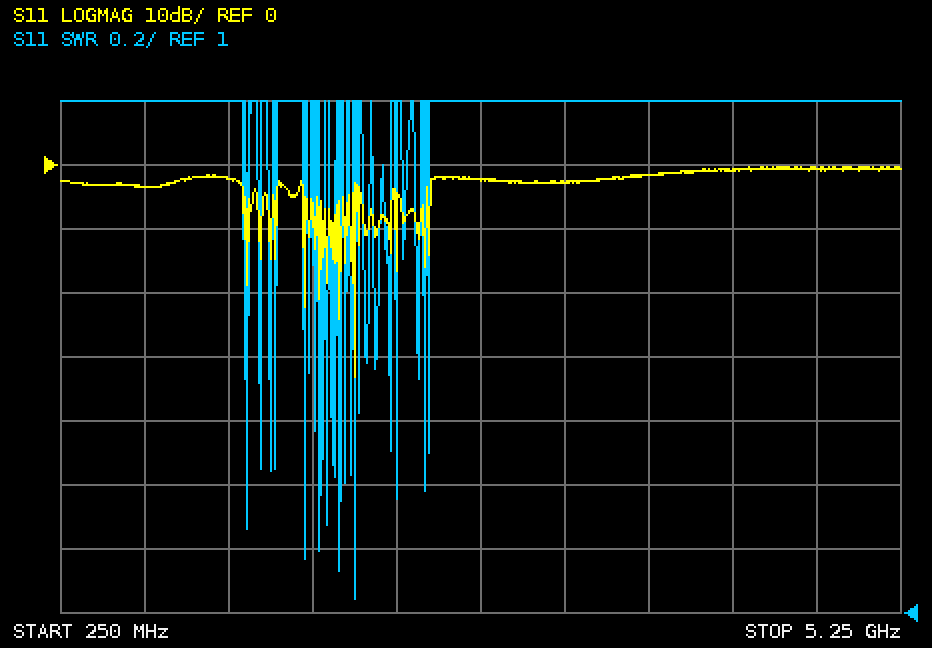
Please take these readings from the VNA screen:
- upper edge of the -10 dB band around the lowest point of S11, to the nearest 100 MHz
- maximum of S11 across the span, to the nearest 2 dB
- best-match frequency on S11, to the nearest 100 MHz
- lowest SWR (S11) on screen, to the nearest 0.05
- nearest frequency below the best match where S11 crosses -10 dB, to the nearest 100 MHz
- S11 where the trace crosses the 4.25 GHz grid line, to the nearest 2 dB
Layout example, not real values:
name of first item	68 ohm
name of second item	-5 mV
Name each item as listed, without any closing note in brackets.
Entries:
upper edge of the -10 dB band around the lowest point of S11, to the nearest 100 MHz	2.0 GHz
maximum of S11 across the span, to the nearest 2 dB	0 dB
best-match frequency on S11, to the nearest 100 MHz	2.0 GHz
lowest SWR (S11) on screen, to the nearest 0.05	1.05
nearest frequency below the best match where S11 crosses -10 dB, to the nearest 100 MHz	2.0 GHz
S11 where the trace crosses the 4.25 GHz grid line, to the nearest 2 dB	0 dB
